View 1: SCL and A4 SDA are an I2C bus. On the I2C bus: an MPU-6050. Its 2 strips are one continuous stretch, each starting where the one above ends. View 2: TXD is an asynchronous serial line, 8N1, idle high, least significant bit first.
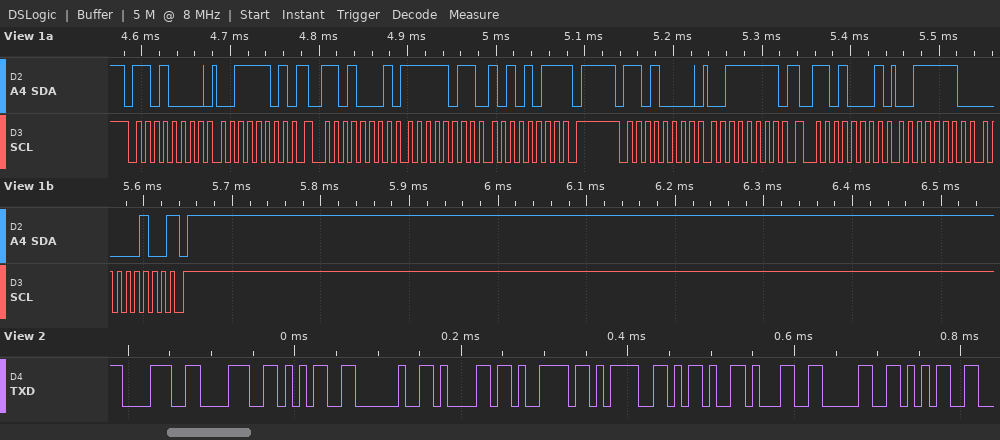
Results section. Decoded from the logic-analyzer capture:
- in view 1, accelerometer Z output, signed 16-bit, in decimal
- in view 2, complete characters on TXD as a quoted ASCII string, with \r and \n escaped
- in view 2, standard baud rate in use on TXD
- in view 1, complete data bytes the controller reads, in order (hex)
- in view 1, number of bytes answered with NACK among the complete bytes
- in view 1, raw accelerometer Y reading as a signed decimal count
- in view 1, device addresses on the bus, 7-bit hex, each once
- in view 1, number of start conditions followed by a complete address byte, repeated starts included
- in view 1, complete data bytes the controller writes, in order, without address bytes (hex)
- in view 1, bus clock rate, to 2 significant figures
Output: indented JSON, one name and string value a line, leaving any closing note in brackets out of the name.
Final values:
{
  "in view 1, accelerometer Z output, signed 16-bit, in decimal": "15876",
  "in view 2, complete characters on TXD as a quoted ASCII string, with \\r and \\n escaped": "\"885 ay=-105\"",
  "in view 2, standard baud rate in use on TXD": "115200 baud",
  "in view 1, complete data bytes the controller reads, in order": "FB AB 3E 04",
  "in view 1, number of bytes answered with NACK among the complete bytes": "2",
  "in view 1, raw accelerometer Y reading as a signed decimal count": "-1109",
  "in view 1, device addresses on the bus, 7-bit hex, each once": "0x68",
  "in view 1, number of start conditions followed by a complete address byte, repeated starts included": "4",
  "in view 1, complete data bytes the controller writes, in order, without address bytes": "3D 3F",
  "in view 1, bus clock rate, to 2 significant figures": "100 kHz"
}
